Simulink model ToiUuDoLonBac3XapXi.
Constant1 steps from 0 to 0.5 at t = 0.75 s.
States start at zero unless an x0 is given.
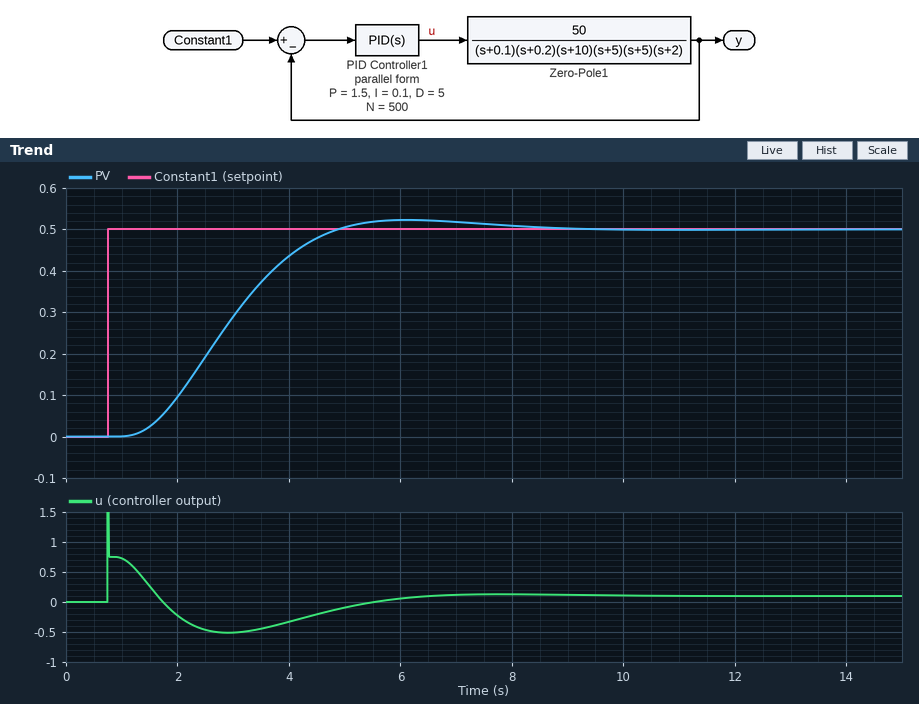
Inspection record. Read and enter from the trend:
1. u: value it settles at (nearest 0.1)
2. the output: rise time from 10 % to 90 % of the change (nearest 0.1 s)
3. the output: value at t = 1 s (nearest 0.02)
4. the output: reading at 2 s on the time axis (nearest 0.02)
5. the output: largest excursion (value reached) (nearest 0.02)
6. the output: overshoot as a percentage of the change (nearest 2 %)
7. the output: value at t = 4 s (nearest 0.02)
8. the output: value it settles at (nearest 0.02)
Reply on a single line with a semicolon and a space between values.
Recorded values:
0.1; 2.4 s; 0.00; 0.10; 0.52; 4 %; 0.44; 0.50
